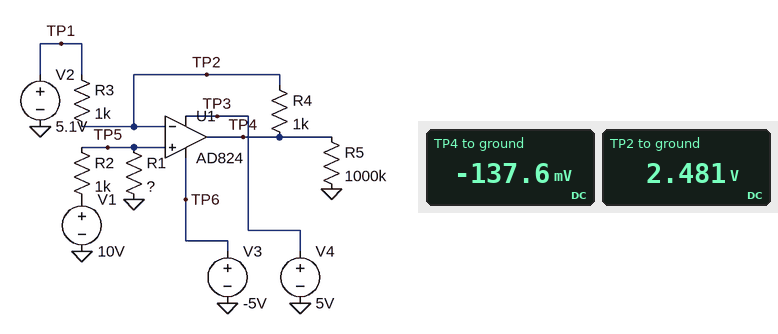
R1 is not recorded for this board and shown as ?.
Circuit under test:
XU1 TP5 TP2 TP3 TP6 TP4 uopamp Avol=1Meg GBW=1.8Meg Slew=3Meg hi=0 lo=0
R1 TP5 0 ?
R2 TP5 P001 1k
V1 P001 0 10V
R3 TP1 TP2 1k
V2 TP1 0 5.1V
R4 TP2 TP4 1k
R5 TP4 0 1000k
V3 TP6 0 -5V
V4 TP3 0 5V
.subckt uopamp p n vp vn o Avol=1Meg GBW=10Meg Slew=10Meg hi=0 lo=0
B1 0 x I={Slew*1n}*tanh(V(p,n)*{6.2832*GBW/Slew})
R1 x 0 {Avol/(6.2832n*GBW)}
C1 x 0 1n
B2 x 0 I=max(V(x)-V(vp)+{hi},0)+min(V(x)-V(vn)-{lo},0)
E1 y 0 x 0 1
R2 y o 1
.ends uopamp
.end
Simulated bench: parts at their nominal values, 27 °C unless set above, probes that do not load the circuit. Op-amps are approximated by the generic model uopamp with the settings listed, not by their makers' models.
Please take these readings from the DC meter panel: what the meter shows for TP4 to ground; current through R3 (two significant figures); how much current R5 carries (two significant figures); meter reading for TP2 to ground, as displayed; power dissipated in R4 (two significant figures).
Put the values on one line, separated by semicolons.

-137.6 mV; 2.6 mA; 140 nA; 2.481 V; 6.9 mW
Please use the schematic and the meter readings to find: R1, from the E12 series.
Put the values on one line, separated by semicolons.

330 Ω
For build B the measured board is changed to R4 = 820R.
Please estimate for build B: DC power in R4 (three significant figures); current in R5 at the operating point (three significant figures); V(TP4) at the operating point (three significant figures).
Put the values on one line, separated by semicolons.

5.62 mW; 334 nA; 334 mV
